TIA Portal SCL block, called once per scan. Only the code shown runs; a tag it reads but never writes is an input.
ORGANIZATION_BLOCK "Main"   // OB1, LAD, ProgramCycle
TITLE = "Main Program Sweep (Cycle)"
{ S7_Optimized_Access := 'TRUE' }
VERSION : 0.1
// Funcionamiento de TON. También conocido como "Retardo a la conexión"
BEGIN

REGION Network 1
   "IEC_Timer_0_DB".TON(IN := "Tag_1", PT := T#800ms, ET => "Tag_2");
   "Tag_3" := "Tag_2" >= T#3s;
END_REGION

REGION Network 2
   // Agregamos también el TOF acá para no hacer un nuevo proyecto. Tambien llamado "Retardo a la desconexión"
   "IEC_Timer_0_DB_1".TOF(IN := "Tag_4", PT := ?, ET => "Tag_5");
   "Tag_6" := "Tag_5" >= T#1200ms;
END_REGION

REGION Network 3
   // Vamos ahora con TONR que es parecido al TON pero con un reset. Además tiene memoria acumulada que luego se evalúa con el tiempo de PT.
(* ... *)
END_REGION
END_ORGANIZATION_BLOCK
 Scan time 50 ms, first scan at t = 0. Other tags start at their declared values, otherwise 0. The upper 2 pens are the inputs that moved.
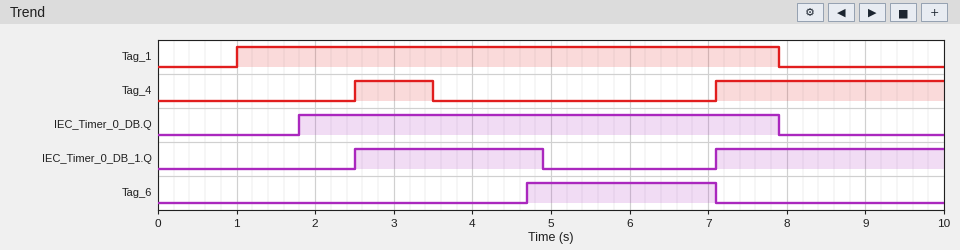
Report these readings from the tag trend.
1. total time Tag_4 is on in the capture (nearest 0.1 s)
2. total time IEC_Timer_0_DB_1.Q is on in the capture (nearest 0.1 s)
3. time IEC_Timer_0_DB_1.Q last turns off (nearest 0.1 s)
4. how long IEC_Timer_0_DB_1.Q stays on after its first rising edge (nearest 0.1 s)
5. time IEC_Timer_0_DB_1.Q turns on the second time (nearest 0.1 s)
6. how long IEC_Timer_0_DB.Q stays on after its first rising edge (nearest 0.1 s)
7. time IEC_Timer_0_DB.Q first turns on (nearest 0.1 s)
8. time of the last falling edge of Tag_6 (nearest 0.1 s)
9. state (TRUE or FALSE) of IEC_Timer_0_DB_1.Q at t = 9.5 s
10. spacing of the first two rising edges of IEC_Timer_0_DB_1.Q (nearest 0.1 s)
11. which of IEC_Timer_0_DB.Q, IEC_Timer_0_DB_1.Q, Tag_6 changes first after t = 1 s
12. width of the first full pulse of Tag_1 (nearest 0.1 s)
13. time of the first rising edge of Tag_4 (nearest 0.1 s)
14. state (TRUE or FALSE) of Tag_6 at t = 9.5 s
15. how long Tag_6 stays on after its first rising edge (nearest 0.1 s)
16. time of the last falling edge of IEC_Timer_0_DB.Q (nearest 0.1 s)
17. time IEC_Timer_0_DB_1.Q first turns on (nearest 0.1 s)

3.9 s
5.3 s
4.9 s
2.4 s
7.1 s
6.1 s
1.8 s
7.1 s
TRUE
4.6 s
IEC_Timer_0_DB.Q
6.9 s
2.5 s
FALSE
2.4 s
7.9 s
2.5 s
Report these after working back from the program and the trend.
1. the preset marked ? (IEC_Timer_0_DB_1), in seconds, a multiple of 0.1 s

1.4 s
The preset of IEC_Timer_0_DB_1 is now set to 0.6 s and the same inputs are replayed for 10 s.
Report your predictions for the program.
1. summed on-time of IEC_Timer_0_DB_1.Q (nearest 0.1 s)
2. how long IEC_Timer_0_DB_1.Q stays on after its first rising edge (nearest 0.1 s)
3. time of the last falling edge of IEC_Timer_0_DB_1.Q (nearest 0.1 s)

4.5 s
1.6 s
4.1 s
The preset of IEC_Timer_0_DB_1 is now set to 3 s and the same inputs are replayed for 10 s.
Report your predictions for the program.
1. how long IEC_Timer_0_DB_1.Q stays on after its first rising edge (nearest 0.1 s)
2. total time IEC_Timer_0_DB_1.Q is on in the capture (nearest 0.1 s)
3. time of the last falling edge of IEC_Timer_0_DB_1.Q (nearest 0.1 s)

4.0 s
6.9 s
6.5 s
